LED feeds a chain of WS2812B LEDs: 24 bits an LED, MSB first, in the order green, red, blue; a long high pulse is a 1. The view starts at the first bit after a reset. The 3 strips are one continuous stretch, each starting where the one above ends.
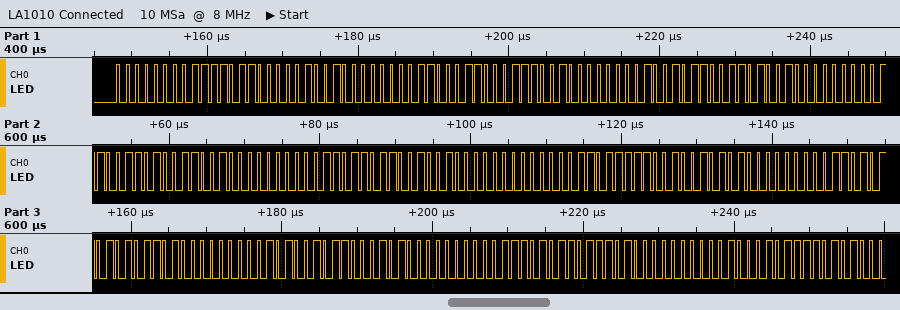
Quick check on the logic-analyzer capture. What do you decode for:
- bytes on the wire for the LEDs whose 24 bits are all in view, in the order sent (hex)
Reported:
00 F6 09 00 C6 39 00 96 69 00 66 99 00 36 C9 00 06 F9 2A 00 D5 5A 00 A5 8A 00 75 BA 00 45
